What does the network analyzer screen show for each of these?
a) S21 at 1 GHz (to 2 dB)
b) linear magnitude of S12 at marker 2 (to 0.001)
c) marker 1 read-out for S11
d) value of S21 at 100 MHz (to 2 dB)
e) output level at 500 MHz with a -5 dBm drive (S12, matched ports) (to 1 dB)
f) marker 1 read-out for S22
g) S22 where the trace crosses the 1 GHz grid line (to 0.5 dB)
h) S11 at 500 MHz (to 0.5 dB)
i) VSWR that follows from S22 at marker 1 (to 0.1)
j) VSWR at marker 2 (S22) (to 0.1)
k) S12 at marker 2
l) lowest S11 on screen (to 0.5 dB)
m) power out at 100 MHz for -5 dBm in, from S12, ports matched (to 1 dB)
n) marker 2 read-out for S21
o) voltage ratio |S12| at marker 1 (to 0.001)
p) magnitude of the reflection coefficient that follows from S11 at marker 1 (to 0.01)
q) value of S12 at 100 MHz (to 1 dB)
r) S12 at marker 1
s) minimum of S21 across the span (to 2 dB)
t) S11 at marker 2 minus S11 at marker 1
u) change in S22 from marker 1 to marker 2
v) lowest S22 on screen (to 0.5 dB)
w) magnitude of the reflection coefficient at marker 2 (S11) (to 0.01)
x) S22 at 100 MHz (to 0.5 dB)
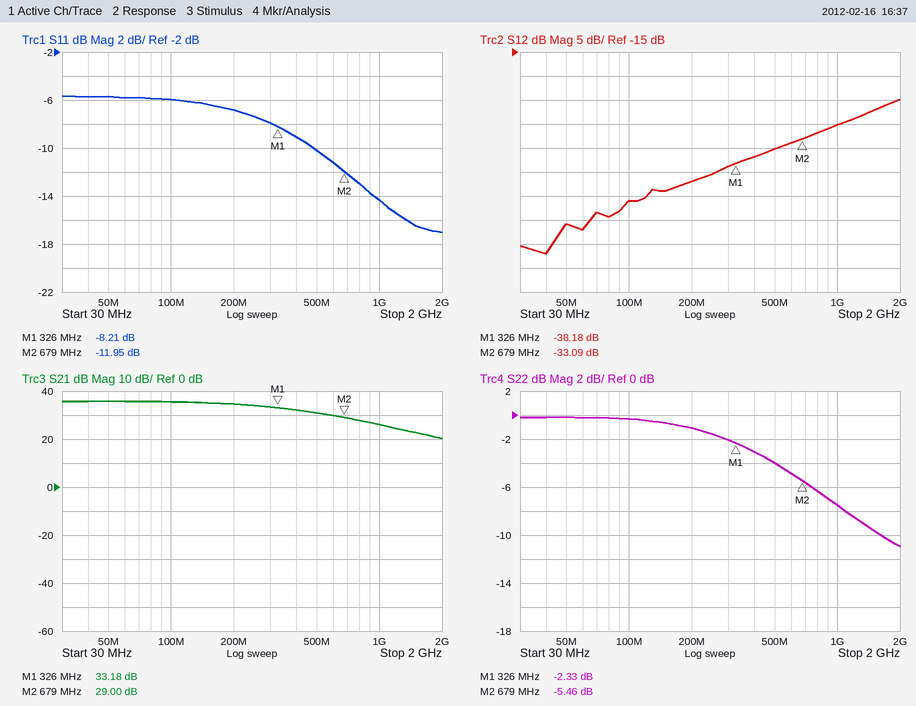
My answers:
26 dB
0.022
-8.21 dB
36 dB
-40 dBm
-2.33 dB
-7.5 dB
-10.0 dB
7.5
3.3
-33.09 dB
-17.0 dB
-51 dBm
29.00 dB
0.012
0.39
-46 dB
-38.18 dB
20 dB
-3.74 dB
-3.13 dB
-11.0 dB
0.25
-0.5 dB
